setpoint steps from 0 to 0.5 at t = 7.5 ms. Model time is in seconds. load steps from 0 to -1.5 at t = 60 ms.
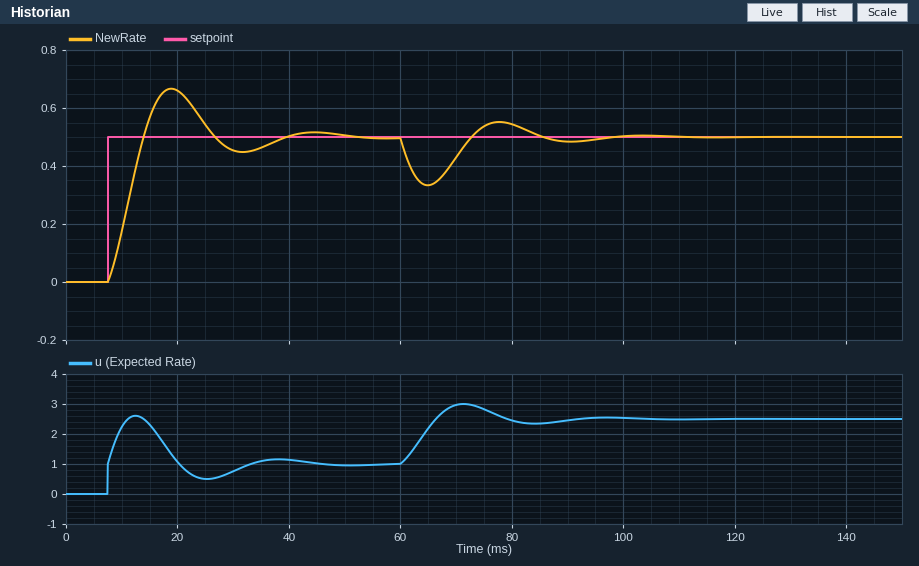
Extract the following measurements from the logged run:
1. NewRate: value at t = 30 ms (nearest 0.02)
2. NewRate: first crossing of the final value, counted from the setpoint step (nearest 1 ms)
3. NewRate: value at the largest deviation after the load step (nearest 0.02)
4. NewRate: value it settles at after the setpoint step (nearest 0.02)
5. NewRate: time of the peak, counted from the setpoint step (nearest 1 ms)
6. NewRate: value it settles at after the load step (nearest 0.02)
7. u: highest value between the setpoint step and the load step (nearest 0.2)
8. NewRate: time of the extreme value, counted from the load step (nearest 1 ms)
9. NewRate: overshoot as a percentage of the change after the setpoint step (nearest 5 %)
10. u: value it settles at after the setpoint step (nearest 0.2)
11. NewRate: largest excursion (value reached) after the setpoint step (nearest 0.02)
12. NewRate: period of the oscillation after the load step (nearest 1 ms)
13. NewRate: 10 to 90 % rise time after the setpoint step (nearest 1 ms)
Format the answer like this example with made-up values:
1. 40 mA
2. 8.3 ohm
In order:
1. 0.46
2. 6 ms
3. 0.34
4. 0.50
5. 11 ms
6. 0.50
7. 2.6
8. 5 ms
9. 35 %
10. 1.0
11. 0.66
12. 26 ms
13. 5 ms
